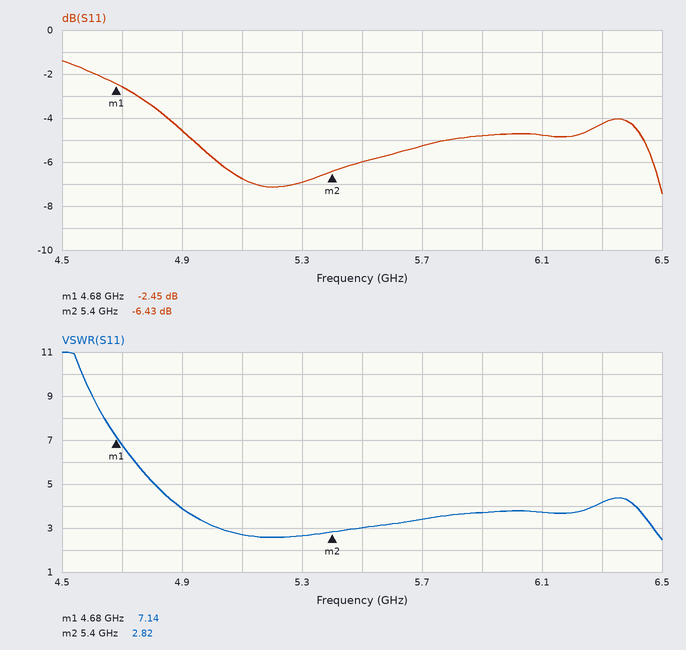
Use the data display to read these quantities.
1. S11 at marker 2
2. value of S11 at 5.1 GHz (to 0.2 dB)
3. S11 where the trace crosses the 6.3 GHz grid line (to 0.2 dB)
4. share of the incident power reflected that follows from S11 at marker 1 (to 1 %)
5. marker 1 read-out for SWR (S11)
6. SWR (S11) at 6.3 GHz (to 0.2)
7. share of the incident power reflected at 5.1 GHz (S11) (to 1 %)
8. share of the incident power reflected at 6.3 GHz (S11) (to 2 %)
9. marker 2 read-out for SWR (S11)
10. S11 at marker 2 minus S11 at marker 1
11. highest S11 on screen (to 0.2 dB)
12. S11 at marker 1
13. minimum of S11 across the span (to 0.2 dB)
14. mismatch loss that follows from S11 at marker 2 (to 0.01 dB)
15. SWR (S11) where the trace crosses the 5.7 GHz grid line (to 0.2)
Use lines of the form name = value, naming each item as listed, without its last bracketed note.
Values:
S11 at marker 2 = -6.43 dB
value of S11 at 5.1 GHz = -6.8 dB
S11 where the trace crosses the 6.3 GHz grid line = -4.2 dB
share of the incident power reflected that follows from S11 at marker 1 = 57 %
marker 1 read-out for SWR = 7.14
SWR (S11) at 6.3 GHz = 4.2
share of the incident power reflected at 5.1 GHz (S11) = 21 %
share of the incident power reflected at 6.3 GHz (S11) = 38 %
marker 2 read-out for SWR = 2.82
S11 at marker 2 minus S11 at marker 1 = -3.98 dB
highest S11 on screen = -1.4 dB
S11 at marker 1 = -2.45 dB
minimum of S11 across the span = -7.4 dB
mismatch loss that follows from S11 at marker 2 = 1.12 dB
SWR (S11) where the trace crosses the 5.7 GHz grid line = 3.4
